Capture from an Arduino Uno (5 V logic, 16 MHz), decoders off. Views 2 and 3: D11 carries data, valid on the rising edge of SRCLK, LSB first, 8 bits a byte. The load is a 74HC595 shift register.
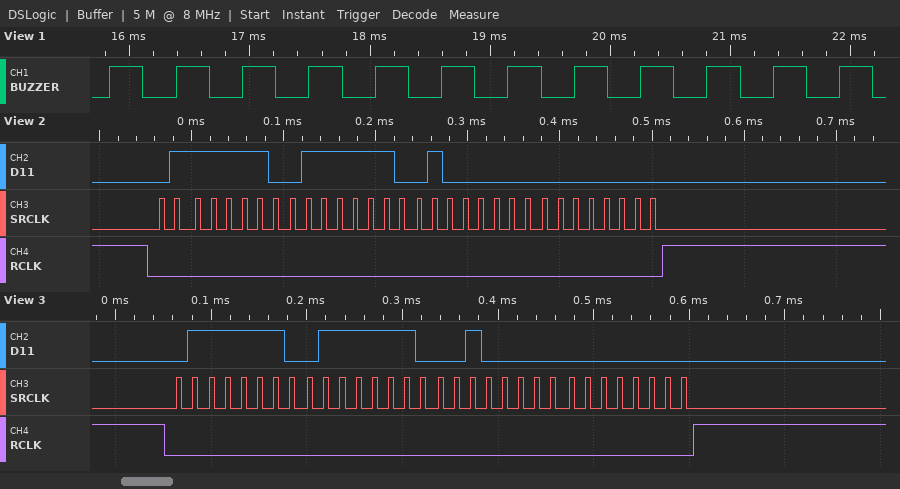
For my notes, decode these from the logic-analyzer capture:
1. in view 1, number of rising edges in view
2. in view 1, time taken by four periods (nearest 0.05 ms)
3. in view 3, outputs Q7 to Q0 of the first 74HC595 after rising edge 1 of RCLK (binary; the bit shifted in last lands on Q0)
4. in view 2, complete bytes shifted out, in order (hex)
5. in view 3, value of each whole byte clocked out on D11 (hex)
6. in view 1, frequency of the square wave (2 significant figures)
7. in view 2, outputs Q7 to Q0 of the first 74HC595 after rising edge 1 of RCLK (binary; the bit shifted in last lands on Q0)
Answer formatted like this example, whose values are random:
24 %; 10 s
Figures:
12; 2.20 ms; 00000000; 0x7E 0x7E 0x02 0x00; 7E 7E 04 00; 1.8 kHz; 00000000
